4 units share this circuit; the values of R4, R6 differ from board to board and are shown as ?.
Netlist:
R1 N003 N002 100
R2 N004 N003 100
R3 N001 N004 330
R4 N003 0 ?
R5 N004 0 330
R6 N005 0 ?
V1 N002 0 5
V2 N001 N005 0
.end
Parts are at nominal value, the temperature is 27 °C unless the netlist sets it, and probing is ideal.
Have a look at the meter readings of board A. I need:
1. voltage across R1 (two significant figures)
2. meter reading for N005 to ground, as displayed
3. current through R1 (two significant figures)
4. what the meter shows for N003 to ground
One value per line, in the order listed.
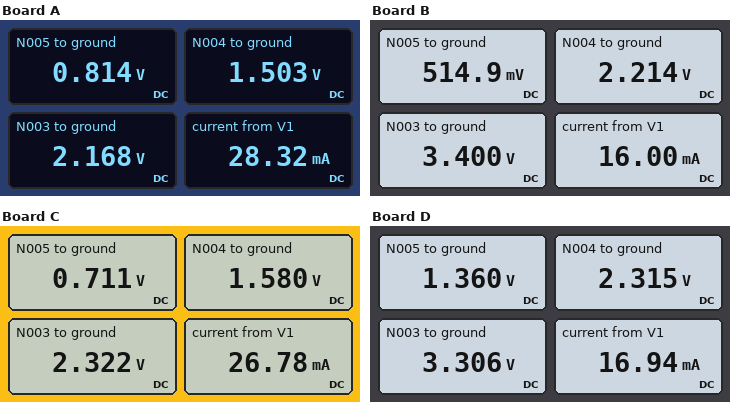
2.8 V
0.814 V
28 mA
2.168 V
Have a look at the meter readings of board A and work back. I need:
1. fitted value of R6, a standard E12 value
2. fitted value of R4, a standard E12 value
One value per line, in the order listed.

390 Ω
100 Ω
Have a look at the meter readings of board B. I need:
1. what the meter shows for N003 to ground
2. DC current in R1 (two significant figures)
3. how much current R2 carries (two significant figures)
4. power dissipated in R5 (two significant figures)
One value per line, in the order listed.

3.400 V
16 mA
12 mA
15 mW
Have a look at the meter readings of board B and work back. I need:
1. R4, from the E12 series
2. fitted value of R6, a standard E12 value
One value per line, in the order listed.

820 Ω
100 Ω
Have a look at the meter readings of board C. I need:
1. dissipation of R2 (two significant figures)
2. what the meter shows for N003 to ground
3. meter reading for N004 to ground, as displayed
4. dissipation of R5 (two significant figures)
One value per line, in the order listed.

5.5 mW
2.322 V
1.580 V
7.6 mW
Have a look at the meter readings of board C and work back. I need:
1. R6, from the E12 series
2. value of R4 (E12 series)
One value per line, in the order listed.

270 Ω
120 Ω
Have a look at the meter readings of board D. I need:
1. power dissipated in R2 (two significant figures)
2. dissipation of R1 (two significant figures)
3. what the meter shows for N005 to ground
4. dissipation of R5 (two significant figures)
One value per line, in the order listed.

9.8 mW
29 mW
1.360 V
16 mW
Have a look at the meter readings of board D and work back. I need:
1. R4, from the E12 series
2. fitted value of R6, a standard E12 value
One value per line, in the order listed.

470 Ω
470 Ω
